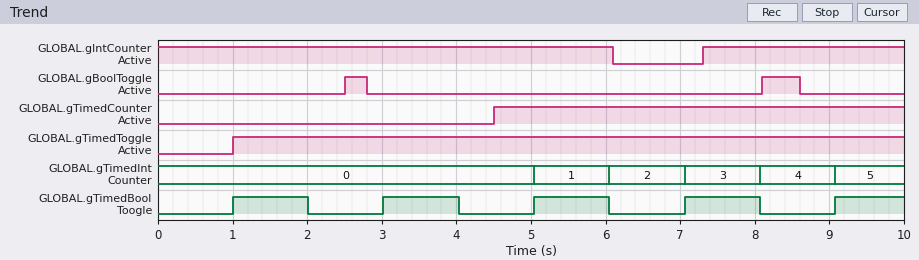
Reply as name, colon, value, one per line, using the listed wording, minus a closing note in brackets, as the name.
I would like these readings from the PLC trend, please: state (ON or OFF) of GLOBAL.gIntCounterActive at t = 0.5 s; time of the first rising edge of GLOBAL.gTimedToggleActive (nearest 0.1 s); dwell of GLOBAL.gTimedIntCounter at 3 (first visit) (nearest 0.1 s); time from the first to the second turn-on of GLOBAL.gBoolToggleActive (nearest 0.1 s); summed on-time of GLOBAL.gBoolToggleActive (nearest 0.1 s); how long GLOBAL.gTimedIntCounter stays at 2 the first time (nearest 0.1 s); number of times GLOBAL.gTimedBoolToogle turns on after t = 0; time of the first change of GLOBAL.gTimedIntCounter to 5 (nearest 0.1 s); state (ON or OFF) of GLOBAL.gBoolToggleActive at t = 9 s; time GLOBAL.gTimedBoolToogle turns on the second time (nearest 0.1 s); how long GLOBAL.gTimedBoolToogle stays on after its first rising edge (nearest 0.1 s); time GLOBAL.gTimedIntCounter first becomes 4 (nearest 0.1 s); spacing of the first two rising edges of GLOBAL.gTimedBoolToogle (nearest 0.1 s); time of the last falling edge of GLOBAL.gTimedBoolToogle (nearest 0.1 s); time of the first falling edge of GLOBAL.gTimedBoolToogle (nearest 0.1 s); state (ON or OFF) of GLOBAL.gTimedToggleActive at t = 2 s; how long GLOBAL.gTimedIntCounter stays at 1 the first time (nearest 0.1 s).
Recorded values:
state (ON or OFF) of GLOBAL.gIntCounterActive at t = 0.5 s: ON
time of the first rising edge of GLOBAL.gTimedToggleActive: 1.0 s
dwell of GLOBAL.gTimedIntCounter at 3 (first visit): 1.0 s
time from the first to the second turn-on of GLOBAL.gBoolToggleActive: 5.6 s
summed on-time of GLOBAL.gBoolToggleActive: 0.8 s
how long GLOBAL.gTimedIntCounter stays at 2 the first time: 1.0 s
number of times GLOBAL.gTimedBoolToogle turns on after t = 0: 5
time of the first change of GLOBAL.gTimedIntCounter to 5: 9.1 s
state (ON or OFF) of GLOBAL.gBoolToggleActive at t = 9 s: OFF
time GLOBAL.gTimedBoolToogle turns on the second time: 3.0 s
how long GLOBAL.gTimedBoolToogle stays on after its first rising edge: 1.0 s
time GLOBAL.gTimedIntCounter first becomes 4: 8.1 s
spacing of the first two rising edges of GLOBAL.gTimedBoolToogle: 2.0 s
time of the last falling edge of GLOBAL.gTimedBoolToogle: 8.1 s
time of the first falling edge of GLOBAL.gTimedBoolToogle: 2.0 s
state (ON or OFF) of GLOBAL.gTimedToggleActive at t = 2 s: ON
how long GLOBAL.gTimedIntCounter stays at 1 the first time: 1.0 s
